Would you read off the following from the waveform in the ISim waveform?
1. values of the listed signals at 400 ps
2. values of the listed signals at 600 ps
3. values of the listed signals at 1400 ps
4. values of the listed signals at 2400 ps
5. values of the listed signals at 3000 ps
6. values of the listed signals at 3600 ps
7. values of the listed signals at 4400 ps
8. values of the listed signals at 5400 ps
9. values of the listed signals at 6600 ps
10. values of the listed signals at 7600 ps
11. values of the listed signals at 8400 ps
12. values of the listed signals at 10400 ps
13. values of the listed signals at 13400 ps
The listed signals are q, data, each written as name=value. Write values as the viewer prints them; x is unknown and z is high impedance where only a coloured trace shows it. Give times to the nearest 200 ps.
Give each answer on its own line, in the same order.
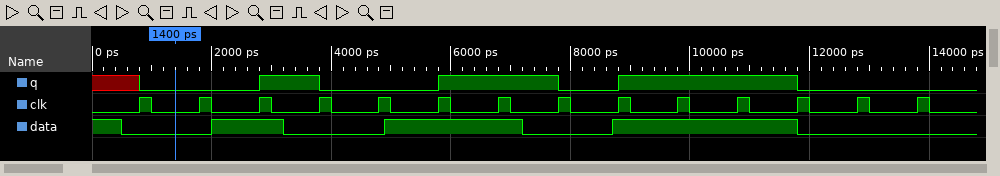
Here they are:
q=x, data=1
q=x, data=0
q=0, data=0
q=0, data=1
q=1, data=1
q=1, data=0
q=0, data=0
q=0, data=1
q=1, data=1
q=1, data=0
q=0, data=0
q=1, data=1
q=0, data=0
